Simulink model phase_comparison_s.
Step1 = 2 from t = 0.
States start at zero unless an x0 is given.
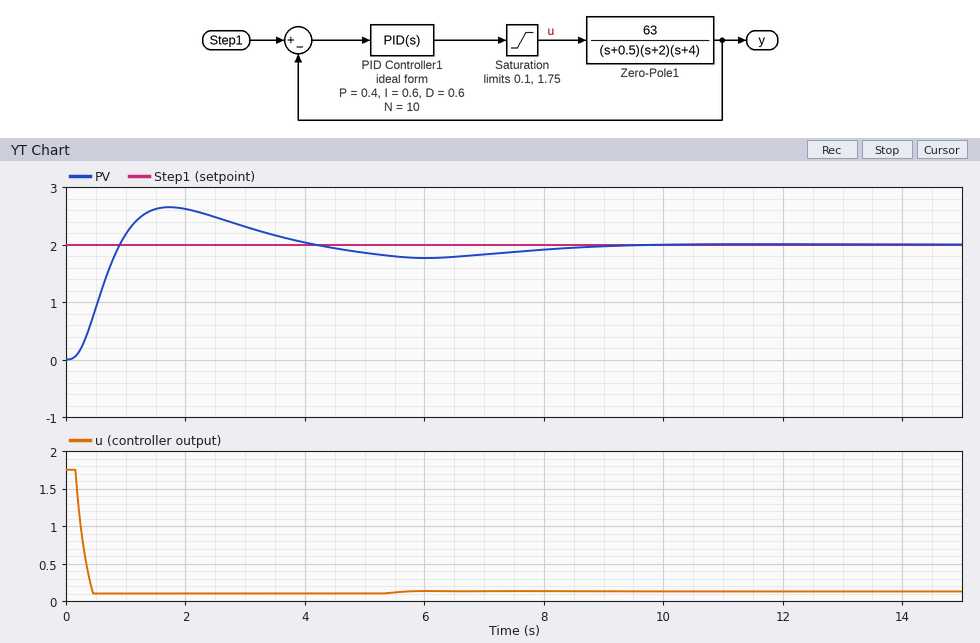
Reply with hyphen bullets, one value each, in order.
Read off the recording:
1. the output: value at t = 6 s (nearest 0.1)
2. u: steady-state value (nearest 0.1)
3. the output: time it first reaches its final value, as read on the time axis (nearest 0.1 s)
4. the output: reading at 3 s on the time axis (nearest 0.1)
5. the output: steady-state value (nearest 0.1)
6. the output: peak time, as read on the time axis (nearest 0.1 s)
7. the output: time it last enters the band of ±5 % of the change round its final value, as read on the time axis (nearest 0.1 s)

- 1.8
- 0.1
- 0.9 s
- 2.3
- 2.0
- 1.7 s
- 7.9 s
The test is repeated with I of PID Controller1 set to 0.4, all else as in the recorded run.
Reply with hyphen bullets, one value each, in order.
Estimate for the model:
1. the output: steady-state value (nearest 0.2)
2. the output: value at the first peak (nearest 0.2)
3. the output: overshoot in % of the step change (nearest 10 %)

- 2.0
- 2.6
- 30 %
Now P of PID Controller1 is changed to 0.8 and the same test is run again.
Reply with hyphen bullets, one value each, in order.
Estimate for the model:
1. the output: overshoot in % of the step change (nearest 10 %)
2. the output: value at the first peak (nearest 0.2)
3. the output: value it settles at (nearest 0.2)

- 60 %
- 3.2
- 2.0
